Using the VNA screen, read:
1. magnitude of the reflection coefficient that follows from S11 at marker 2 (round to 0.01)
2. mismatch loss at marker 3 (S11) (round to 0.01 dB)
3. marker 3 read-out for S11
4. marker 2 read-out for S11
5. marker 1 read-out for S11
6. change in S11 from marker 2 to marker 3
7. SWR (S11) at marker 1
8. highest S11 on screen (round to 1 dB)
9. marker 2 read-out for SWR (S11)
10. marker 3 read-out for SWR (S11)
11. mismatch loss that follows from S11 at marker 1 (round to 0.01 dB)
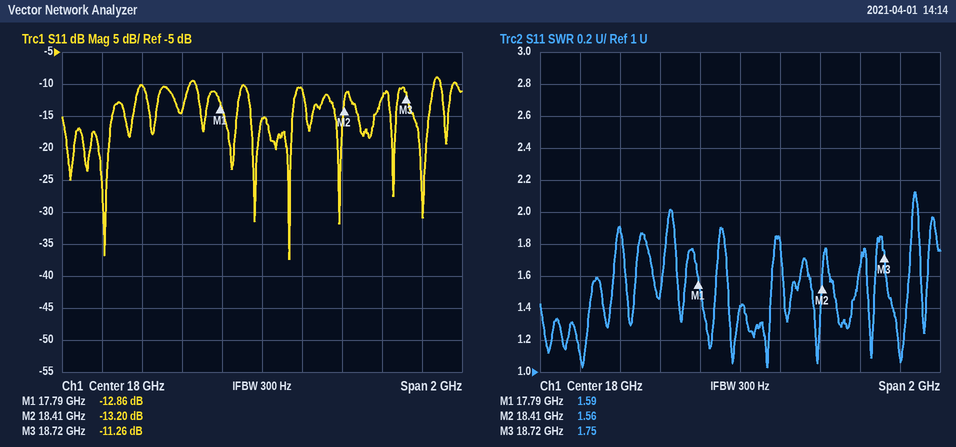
0.22
0.34 dB
-11.26 dB
-13.20 dB
-12.86 dB
1.94 dB
1.59
-9 dB
1.56
1.75
0.23 dB
